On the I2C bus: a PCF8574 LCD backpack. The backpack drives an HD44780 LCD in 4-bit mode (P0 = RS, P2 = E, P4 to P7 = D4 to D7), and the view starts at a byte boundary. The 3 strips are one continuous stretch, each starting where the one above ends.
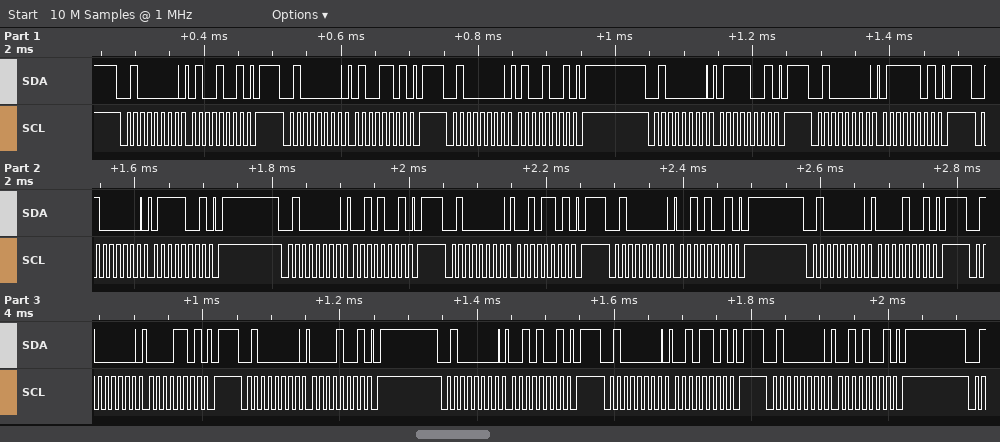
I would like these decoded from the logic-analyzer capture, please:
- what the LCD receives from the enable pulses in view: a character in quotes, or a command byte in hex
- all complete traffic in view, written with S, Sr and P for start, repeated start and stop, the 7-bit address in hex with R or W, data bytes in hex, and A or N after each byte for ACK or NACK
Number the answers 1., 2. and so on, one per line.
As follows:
1. 'G' ' '
2. S 20W A 49 A P S 20W A 4D A P S 20W A 49 A P S 20W A 79 A P S 20W A 7D A P S 20W A 79 A P S 20W A 29 A P S 20W A 2D A P S 20W A 29 A P S 20W A 09 A P S 20W A 0D A P S 20W A 09 A P S 20W A 29 A P S 20W A 2D A P S 20W A 29 A P
